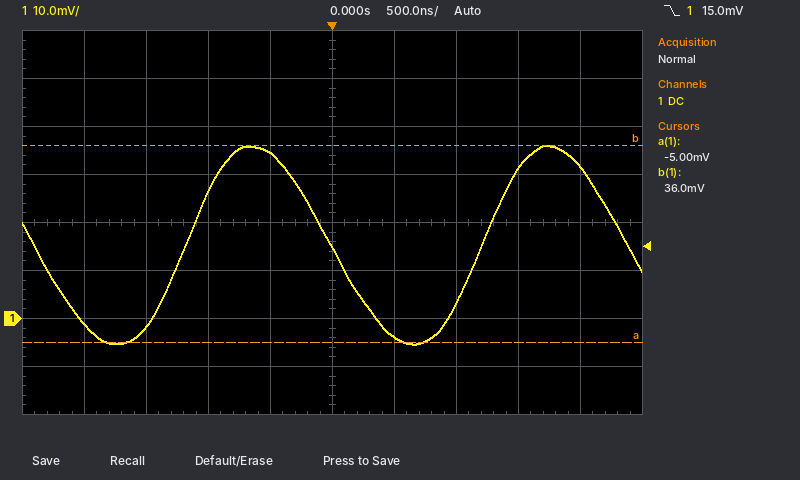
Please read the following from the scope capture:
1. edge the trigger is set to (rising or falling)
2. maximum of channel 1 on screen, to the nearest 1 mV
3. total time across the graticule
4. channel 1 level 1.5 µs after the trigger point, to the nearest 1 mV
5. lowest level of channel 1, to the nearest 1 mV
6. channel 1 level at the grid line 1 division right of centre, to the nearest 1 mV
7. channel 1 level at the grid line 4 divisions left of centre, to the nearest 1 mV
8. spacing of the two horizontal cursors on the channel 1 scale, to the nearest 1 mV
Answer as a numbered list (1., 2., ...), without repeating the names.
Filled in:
1. falling
2. 36 mV
3. 5 µs
4. 31 mV
5. -5 mV
6. -4 mV
7. -1 mV
8. 41 mV
